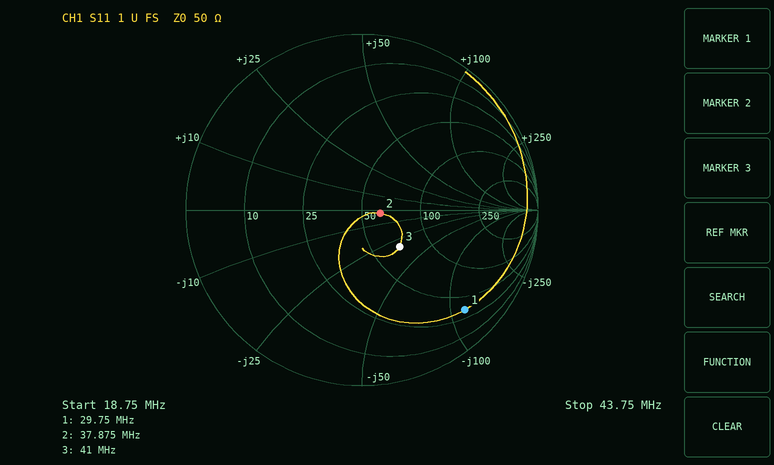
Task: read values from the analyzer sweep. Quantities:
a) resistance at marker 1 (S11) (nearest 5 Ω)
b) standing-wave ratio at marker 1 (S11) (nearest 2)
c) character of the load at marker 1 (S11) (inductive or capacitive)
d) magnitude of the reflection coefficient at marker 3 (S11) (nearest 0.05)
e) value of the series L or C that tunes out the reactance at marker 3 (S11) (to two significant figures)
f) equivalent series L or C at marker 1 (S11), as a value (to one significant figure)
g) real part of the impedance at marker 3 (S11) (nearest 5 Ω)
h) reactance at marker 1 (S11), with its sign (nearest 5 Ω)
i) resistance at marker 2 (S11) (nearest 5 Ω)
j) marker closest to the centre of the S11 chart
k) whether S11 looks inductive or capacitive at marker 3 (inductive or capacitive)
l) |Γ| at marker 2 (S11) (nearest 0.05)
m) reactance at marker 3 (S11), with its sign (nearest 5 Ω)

35 Ω
10
capacitive
0.30
120 nH
50 pF
70 Ω
-115 Ω
60 Ω
marker 2
capacitive
0.10
-30 Ω
